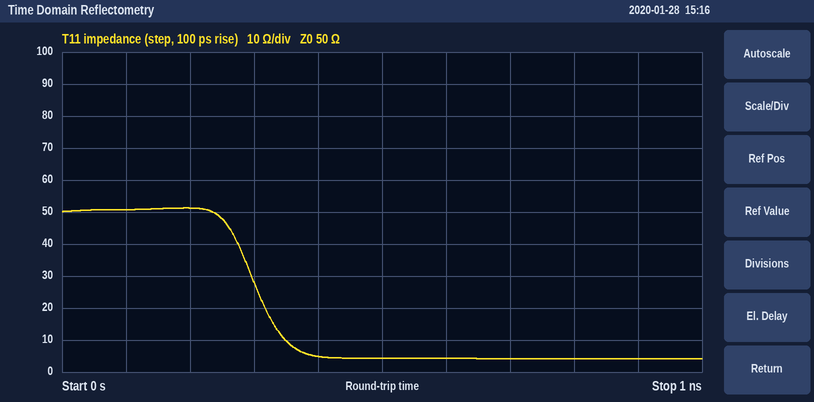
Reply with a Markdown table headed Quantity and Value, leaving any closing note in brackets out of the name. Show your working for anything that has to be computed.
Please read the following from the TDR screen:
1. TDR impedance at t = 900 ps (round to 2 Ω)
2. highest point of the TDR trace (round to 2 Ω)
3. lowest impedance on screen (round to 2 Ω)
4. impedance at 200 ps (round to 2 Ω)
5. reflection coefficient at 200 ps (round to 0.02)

| Quantity | Value |
|---|---|
| TDR impedance at t = 900 ps | 4 Ω |
| highest point of the TDR trace | 52 Ω |
| lowest impedance on screen | 4 Ω |
| impedance at 200 ps | 52 Ω |
| reflection coefficient at 200 ps | (52 − 50)/(52 + 50) ≈ +0.02 |
